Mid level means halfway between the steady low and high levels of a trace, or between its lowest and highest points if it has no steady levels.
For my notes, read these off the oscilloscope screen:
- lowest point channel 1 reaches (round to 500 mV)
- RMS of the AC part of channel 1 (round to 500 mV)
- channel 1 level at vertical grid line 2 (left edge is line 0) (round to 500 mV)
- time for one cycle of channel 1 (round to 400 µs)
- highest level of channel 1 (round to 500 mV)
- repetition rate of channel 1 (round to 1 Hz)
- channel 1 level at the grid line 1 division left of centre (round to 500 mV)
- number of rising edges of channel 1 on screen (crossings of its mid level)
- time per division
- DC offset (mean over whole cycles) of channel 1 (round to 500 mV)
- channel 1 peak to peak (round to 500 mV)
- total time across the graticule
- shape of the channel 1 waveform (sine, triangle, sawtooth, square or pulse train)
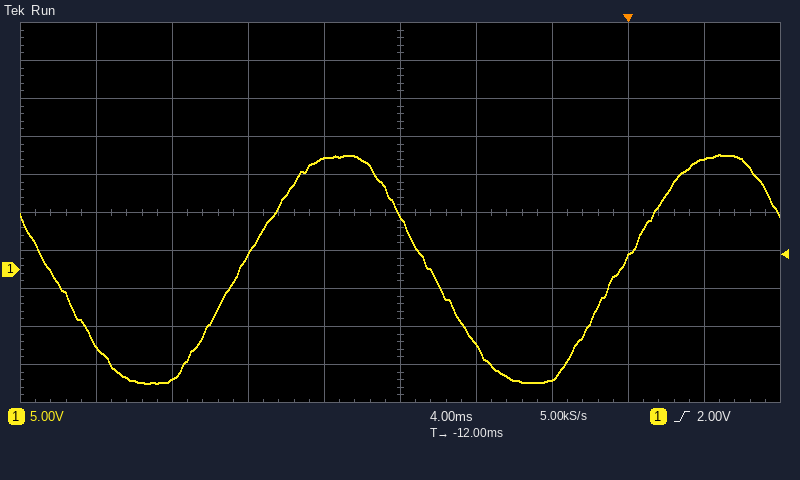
-15.0 V
10.5 V
-14.5 V
20.0 ms
15.0 V
50 Hz
14.5 V
2
4 ms
0.0 V
30.0 V
40 ms
sine
